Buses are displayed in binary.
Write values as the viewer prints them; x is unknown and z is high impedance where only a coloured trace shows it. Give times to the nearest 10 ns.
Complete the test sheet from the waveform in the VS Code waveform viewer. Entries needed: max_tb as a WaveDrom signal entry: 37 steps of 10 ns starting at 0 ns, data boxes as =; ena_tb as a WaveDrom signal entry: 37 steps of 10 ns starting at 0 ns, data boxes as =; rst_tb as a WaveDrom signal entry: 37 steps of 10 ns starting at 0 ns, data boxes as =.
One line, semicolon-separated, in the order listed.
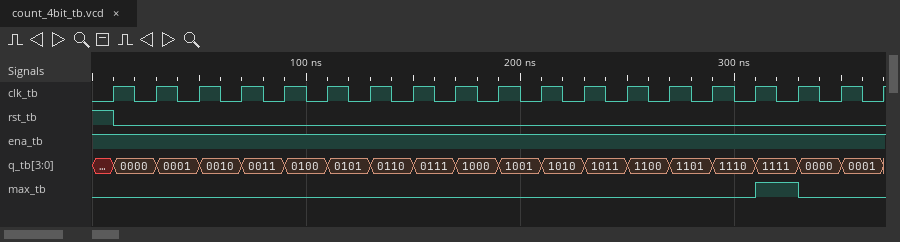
{name: 'max_tb', wave: '0..............................1.0...'}; {name: 'ena_tb', wave: '1....................................'}; {name: 'rst_tb', wave: '10...................................'}
